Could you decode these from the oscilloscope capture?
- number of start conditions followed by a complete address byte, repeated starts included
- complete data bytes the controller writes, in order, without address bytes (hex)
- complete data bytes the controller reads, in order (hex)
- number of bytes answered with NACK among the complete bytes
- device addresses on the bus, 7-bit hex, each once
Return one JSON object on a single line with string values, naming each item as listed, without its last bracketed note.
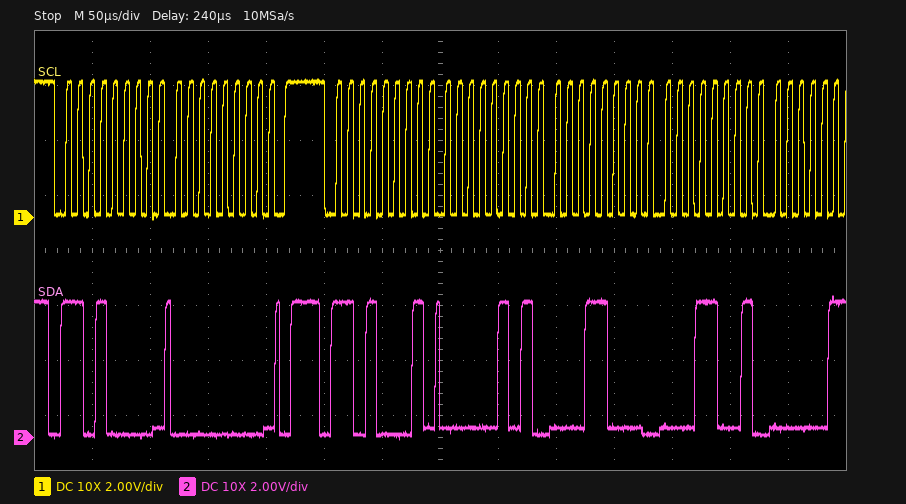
{"number of start conditions followed by a complete address byte, repeated starts included": "2", "complete data bytes the controller writes, in order, without address bytes": "00", "complete data bytes the controller reads, in order": "05 18 19", "number of bytes answered with NACK among the complete bytes": "0", "device addresses on the bus, 7-bit hex, each once": "0x68"}
